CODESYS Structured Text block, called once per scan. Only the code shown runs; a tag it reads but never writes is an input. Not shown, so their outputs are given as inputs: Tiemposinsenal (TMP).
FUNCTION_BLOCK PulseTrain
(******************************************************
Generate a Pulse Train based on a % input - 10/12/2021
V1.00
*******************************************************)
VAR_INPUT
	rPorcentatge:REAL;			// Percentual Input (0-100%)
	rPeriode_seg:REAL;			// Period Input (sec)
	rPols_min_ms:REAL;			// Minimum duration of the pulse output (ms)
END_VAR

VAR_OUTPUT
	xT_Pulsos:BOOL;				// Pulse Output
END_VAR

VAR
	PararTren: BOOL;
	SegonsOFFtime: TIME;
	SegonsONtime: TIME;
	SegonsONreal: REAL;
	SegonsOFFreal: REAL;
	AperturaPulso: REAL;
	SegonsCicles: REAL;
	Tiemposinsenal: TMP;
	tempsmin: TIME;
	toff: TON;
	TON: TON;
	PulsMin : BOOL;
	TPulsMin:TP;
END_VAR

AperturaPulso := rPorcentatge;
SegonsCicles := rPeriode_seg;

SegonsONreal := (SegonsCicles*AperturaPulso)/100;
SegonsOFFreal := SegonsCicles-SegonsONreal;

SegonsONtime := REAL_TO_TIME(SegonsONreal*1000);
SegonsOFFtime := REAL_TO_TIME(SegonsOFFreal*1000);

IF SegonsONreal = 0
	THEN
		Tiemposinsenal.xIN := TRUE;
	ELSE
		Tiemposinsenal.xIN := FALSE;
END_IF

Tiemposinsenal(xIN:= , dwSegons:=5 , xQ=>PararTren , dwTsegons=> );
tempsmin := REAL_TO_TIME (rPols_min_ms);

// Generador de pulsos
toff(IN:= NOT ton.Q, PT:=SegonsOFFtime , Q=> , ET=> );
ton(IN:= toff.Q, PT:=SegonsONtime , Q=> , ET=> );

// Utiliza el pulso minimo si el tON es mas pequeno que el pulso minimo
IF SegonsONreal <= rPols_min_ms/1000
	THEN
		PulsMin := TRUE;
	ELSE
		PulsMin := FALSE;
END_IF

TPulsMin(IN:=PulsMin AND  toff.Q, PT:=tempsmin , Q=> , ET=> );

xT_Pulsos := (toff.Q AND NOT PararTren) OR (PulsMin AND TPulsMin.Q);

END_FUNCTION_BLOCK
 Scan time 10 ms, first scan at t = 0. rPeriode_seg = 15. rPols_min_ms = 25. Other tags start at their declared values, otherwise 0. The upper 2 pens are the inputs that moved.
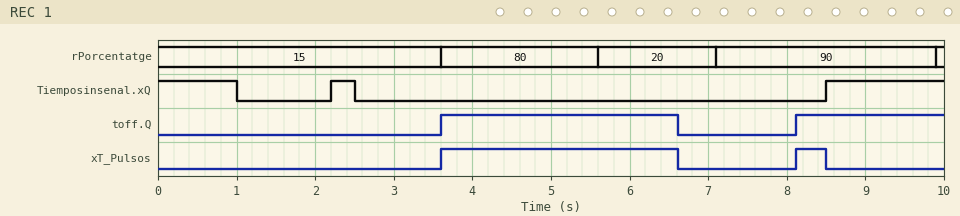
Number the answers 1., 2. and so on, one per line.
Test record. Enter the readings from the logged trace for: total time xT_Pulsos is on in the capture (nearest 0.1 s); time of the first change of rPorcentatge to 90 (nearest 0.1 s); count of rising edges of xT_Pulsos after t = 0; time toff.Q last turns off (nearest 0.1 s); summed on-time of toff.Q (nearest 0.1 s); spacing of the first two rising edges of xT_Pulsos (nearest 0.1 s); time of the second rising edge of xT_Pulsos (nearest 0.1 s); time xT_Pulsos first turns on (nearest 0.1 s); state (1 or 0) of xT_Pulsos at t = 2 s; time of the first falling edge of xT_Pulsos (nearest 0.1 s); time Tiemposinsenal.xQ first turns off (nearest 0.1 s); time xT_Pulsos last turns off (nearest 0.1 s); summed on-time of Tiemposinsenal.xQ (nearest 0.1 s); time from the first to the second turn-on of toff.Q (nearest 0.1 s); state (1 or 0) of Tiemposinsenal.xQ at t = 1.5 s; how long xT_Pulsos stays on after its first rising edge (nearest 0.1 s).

1. 3.4 s
2. 7.1 s
3. 2
4. 6.6 s
5. 4.9 s
6. 4.5 s
7. 8.1 s
8. 3.6 s
9. 0
10. 6.6 s
11. 1.0 s
12. 8.5 s
13. 2.8 s
14. 4.5 s
15. 0
16. 3.0 s
